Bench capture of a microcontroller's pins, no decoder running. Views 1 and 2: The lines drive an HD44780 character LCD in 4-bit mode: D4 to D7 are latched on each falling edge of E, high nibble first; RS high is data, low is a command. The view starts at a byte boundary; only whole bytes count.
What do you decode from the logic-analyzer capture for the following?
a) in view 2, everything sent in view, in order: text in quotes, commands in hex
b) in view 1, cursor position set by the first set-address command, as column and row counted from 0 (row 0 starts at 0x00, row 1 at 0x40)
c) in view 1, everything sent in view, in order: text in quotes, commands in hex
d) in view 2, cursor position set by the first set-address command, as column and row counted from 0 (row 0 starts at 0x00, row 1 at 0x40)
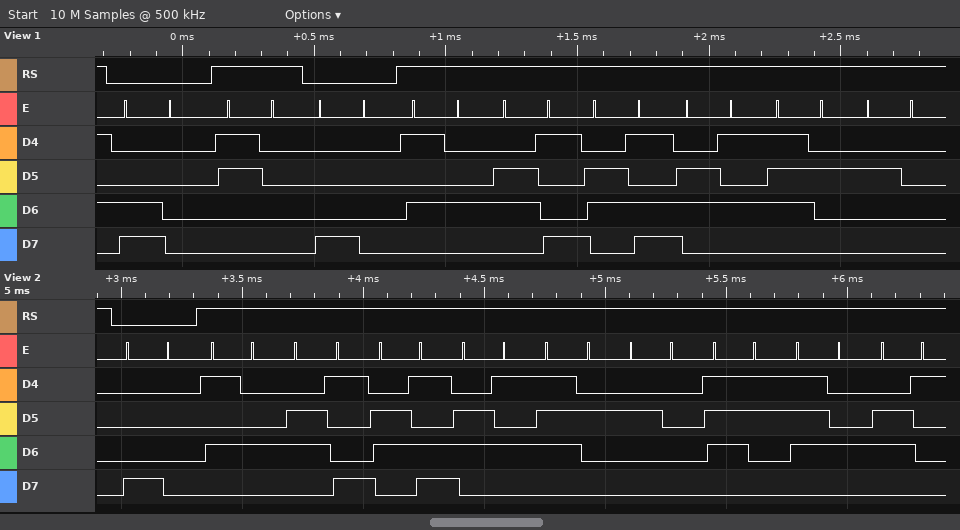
0x80 "Timer sta"
column 0, row 1
0xC0 "0" 0x80 "Timer "
column 0, row 0
